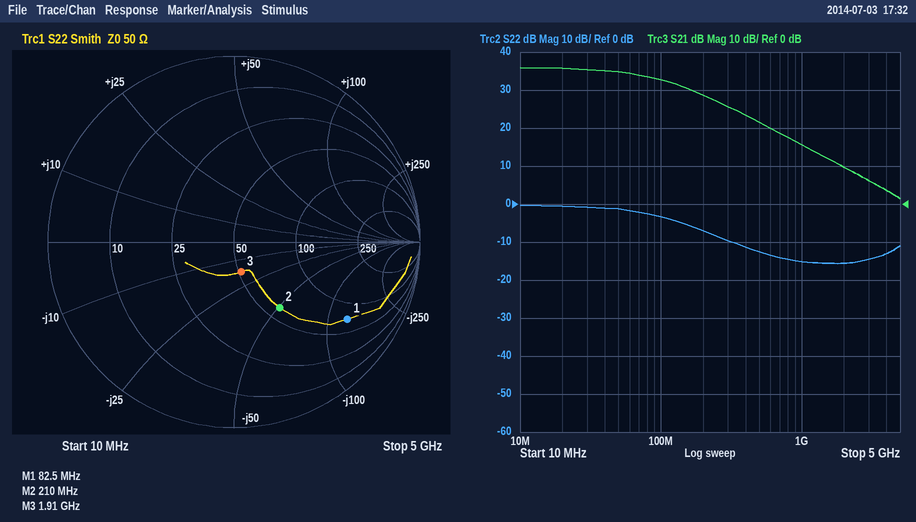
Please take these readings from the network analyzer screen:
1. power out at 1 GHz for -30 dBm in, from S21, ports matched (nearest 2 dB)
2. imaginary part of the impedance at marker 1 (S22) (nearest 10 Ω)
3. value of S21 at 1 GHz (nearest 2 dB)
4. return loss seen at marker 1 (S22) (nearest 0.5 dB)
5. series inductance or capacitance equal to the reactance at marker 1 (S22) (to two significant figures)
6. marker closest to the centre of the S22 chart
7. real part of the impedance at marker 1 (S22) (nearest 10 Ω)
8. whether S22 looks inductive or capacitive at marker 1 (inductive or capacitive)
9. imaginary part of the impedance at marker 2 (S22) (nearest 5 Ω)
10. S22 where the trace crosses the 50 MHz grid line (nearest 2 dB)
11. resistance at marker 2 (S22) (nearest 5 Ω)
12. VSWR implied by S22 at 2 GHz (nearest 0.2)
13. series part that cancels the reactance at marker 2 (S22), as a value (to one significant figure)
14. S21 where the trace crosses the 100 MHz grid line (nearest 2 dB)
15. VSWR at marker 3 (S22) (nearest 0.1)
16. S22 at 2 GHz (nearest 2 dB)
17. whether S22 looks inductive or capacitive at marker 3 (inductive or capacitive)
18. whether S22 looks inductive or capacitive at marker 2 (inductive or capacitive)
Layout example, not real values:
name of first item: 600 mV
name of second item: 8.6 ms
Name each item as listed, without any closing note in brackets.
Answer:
power out at 1 GHz for -30 dBm in, from S21, ports matched: -14 dBm
imaginary part of the impedance at marker 1 (S22): -130 Ω
value of S21 at 1 GHz: 16 dB
return loss seen at marker 1 (S22): 2.5 dB
series inductance or capacitance equal to the reactance at marker 1 (S22): 15 pF
marker closest to the centre of the S22 chart: marker 3
real part of the impedance at marker 1 (S22): 70 Ω
whether S22 looks inductive or capacitive at marker 1: capacitive
imaginary part of the impedance at marker 2 (S22): -50 Ω
S22 where the trace crosses the 50 MHz grid line: -2 dB
resistance at marker 2 (S22): 60 Ω
VSWR implied by S22 at 2 GHz: 1.4
series part that cancels the reactance at marker 2 (S22), as a value: 40 nH
S21 where the trace crosses the 100 MHz grid line: 32 dB
VSWR at marker 3 (S22): 1.4
S22 at 2 GHz: -16 dB
whether S22 looks inductive or capacitive at marker 3: capacitive
whether S22 looks inductive or capacitive at marker 2: capacitive
